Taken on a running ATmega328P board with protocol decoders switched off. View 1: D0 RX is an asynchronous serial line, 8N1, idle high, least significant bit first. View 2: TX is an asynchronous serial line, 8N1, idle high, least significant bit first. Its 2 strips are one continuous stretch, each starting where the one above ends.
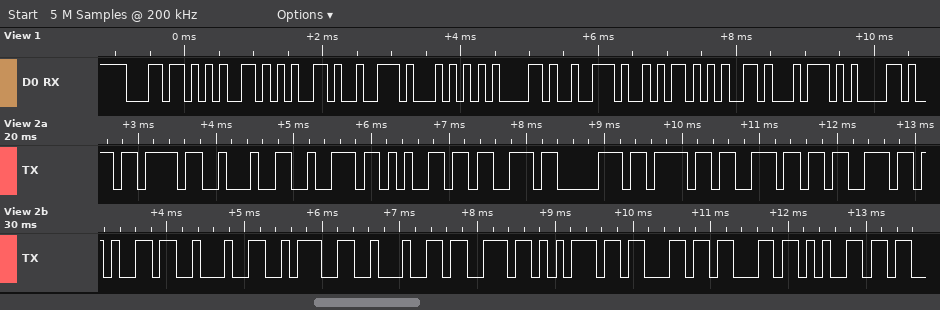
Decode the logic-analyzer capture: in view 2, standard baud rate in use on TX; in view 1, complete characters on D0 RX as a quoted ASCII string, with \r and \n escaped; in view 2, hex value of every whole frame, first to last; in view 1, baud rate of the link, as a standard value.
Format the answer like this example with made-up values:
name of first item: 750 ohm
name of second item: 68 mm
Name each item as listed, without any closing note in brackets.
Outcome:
in view 2, standard baud rate in use on TX: 9600 baud
in view 1, complete characters on D0 RX as a quoted ASCII string, with \r and \n escaped: "leerTarjeta"
in view 2, hex value of every whole frame, first to last: 7B 22 72 65 73 70 6F 6E 73 65 22 3A 22 73 75 63 63 65
in view 1, baud rate of the link, as a standard value: 9600 baud
